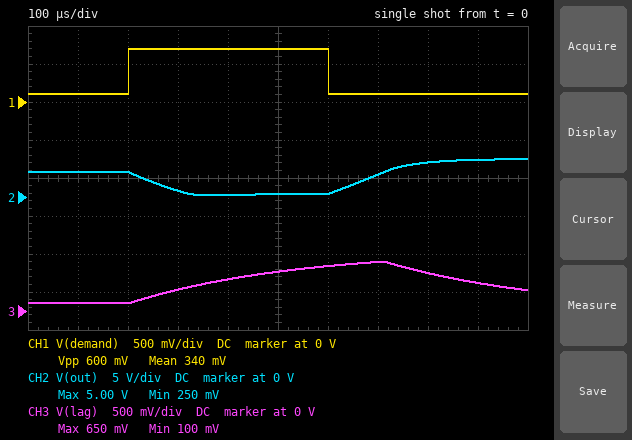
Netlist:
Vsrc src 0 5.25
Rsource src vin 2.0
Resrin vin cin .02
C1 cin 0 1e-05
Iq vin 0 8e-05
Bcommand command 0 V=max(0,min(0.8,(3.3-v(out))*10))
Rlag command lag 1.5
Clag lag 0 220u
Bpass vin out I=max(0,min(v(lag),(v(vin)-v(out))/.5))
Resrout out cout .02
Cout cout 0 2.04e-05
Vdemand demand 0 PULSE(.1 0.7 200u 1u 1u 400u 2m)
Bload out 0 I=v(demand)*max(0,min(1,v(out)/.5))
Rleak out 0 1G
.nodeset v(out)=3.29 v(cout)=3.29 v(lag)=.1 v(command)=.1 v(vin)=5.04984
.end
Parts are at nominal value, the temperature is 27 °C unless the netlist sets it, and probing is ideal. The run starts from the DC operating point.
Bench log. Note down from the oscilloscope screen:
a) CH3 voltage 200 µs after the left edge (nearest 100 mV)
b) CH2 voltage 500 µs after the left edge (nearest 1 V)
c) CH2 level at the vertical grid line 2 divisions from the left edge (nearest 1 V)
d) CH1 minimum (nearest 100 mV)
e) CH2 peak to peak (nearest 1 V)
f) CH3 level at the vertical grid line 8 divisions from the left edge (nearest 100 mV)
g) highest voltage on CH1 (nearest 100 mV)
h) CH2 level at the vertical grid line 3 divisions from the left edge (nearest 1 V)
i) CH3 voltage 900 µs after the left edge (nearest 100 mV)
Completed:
100 mV
0 V
3 V
100 mV
5 V
500 mV
700 mV
1 V
400 mV
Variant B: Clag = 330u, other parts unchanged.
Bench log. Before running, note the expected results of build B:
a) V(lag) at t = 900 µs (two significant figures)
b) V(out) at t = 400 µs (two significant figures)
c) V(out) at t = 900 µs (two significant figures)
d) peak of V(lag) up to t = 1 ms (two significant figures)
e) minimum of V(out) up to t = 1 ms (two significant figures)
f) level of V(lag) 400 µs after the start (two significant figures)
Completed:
410 mV
230 mV
4.8 V
560 mV
210 mV
330 mV
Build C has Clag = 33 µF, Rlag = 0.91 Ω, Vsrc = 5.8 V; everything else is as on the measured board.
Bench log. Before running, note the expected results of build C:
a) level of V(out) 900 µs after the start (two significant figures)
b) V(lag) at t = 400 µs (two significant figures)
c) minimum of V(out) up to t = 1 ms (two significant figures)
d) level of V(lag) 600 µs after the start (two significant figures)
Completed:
3.3 V
800 mV
2.7 V
700 mV
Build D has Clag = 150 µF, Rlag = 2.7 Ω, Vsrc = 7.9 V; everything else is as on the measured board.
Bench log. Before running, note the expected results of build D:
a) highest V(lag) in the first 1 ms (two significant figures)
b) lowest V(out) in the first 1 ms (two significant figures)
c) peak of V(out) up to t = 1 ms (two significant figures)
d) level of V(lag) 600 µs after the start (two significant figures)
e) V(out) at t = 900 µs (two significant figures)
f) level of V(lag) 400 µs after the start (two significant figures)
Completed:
610 mV
230 mV
7.4 V
540 mV
6.6 V
370 mV
